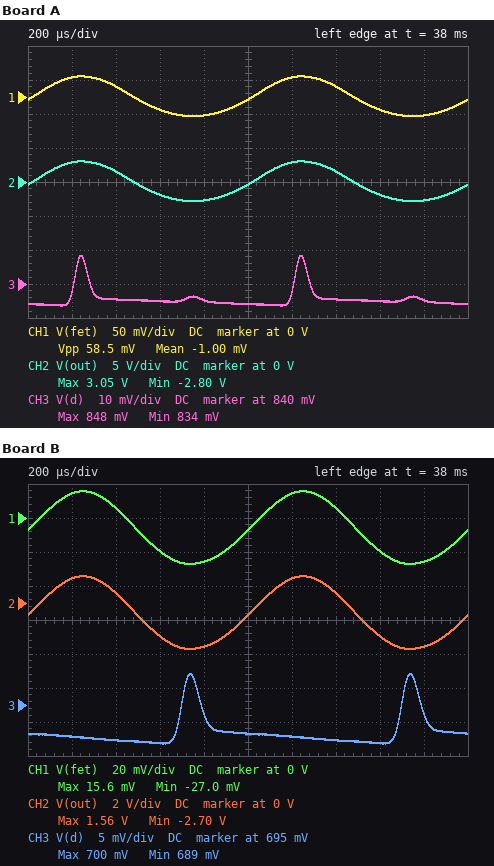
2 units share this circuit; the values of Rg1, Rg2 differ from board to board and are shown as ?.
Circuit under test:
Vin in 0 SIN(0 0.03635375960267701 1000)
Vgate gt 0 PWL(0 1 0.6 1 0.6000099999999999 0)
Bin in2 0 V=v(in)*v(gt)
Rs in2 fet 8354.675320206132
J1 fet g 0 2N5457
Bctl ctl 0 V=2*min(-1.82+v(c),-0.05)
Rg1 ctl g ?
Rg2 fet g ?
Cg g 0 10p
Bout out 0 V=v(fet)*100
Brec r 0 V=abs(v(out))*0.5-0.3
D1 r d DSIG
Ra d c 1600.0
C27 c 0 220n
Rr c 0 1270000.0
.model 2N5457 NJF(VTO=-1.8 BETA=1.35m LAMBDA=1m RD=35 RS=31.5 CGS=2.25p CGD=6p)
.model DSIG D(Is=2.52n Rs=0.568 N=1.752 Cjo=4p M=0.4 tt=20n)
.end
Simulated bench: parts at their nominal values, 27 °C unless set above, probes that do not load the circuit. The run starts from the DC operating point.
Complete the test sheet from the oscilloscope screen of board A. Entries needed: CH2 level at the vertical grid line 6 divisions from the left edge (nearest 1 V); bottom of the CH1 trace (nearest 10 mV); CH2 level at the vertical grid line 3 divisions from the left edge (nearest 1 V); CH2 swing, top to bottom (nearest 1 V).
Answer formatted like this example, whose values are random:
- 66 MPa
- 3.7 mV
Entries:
- 3 V
- -30 mV
- -2 V
- 6 V
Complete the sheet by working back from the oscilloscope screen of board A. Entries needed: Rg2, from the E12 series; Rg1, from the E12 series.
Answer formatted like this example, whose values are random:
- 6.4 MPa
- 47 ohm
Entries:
- 3.3 MΩ
- 330 kΩ
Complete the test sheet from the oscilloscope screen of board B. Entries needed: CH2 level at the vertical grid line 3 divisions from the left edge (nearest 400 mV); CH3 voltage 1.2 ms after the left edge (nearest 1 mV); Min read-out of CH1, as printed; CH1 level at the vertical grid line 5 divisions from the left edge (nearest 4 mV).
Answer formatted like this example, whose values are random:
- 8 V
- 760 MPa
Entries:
- -2.0 V
- 690 mV
- -27.0 mV
- -8 mV
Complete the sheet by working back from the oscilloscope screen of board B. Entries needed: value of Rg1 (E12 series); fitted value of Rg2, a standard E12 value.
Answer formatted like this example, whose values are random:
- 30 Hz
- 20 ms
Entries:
- 330 kΩ
- 1.2 MΩ
